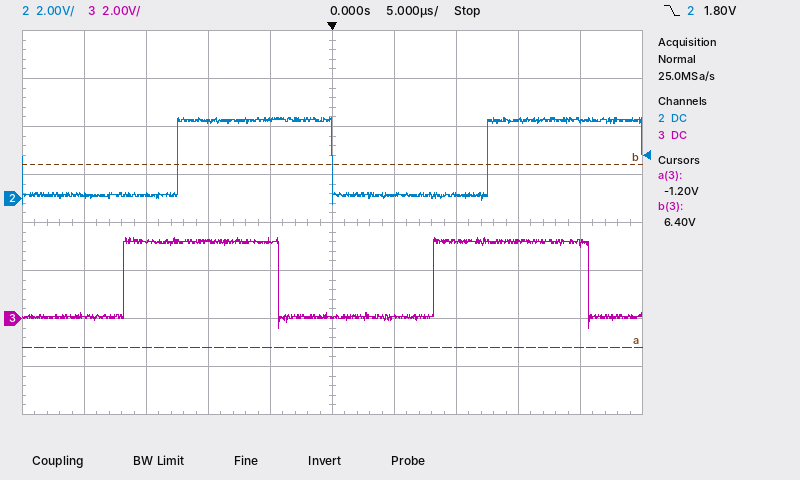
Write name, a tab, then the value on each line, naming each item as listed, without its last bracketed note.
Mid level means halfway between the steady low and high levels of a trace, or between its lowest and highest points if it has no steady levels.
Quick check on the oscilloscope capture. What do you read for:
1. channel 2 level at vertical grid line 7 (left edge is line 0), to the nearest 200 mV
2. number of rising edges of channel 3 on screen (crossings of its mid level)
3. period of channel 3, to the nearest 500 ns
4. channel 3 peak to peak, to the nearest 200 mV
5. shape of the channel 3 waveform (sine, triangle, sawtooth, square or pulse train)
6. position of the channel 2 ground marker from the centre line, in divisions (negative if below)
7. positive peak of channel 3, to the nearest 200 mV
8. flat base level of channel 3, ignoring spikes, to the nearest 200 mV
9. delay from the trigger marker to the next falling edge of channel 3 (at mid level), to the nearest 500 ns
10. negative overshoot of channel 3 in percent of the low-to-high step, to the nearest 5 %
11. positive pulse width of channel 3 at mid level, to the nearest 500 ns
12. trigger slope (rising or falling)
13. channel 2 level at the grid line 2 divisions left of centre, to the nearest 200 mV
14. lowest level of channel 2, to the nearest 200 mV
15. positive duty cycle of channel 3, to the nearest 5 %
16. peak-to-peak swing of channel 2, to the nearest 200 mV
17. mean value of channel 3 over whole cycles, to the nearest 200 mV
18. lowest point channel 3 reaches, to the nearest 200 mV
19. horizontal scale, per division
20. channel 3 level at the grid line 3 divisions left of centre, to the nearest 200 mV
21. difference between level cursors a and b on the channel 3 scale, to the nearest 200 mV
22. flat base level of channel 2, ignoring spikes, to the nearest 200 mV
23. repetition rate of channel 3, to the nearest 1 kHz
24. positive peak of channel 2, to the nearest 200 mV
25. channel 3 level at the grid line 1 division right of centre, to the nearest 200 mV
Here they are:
channel 2 level at vertical grid line 7 (left edge is line 0), to the nearest 200 mV	200 mV
number of rising edges of channel 3 on screen	2
period of channel 3, to the nearest 500 ns	25.0 µs
channel 3 peak to peak, to the nearest 200 mV	3.8 V
shape of the channel 3 waveform	square
position of the channel 2 ground marker from the centre line, in divisions	+0.5 div
positive peak of channel 3, to the nearest 200 mV	3.4 V
flat base level of channel 3, ignoring spikes, to the nearest 200 mV	0.0 V
delay from the trigger marker to the next falling edge of channel 3 (at mid level), to the nearest 500 ns	20.5 µs
negative overshoot of channel 3 in percent of the low-to-high step, to the nearest 5 %	15 %
positive pulse width of channel 3 at mid level, to the nearest 500 ns	12.5 µs
trigger slope	falling
channel 2 level at the grid line 2 divisions left of centre, to the nearest 200 mV	3.2 V
lowest level of channel 2, to the nearest 200 mV	-200 mV
positive duty cycle of channel 3, to the nearest 5 %	50 %
peak-to-peak swing of channel 2, to the nearest 200 mV	3.6 V
mean value of channel 3 over whole cycles, to the nearest 200 mV	1.6 V
lowest point channel 3 reaches, to the nearest 200 mV	-400 mV
horizontal scale, per division	5 µs
channel 3 level at the grid line 3 divisions left of centre, to the nearest 200 mV	3.2 V
difference between level cursors a and b on the channel 3 scale, to the nearest 200 mV	7.6 V
flat base level of channel 2, ignoring spikes, to the nearest 200 mV	200 mV
repetition rate of channel 3, to the nearest 1 kHz	40 kHz
positive peak of channel 2, to the nearest 200 mV	3.4 V
channel 3 level at the grid line 1 division right of centre, to the nearest 200 mV	0.0 V
